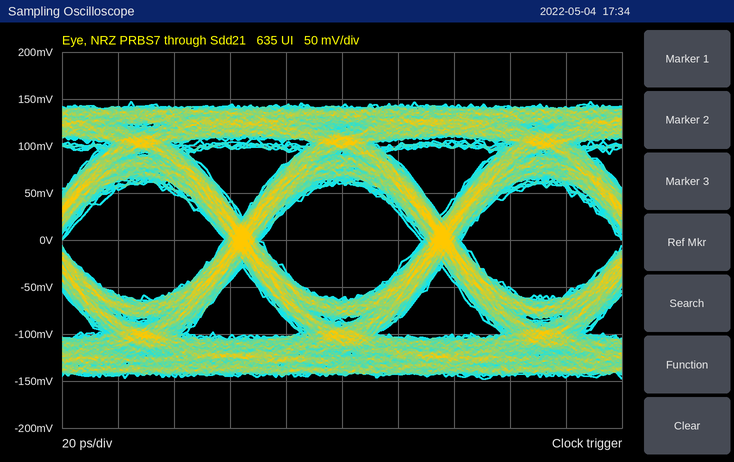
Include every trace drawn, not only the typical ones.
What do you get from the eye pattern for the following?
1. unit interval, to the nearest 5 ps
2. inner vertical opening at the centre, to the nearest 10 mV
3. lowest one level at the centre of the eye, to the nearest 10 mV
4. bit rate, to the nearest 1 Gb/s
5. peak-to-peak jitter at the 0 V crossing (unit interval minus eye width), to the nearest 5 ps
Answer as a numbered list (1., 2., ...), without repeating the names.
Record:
1. 70 ps
2. 120 mV
3. 60 mV
4. 14 Gb/s
5. 15 ps
